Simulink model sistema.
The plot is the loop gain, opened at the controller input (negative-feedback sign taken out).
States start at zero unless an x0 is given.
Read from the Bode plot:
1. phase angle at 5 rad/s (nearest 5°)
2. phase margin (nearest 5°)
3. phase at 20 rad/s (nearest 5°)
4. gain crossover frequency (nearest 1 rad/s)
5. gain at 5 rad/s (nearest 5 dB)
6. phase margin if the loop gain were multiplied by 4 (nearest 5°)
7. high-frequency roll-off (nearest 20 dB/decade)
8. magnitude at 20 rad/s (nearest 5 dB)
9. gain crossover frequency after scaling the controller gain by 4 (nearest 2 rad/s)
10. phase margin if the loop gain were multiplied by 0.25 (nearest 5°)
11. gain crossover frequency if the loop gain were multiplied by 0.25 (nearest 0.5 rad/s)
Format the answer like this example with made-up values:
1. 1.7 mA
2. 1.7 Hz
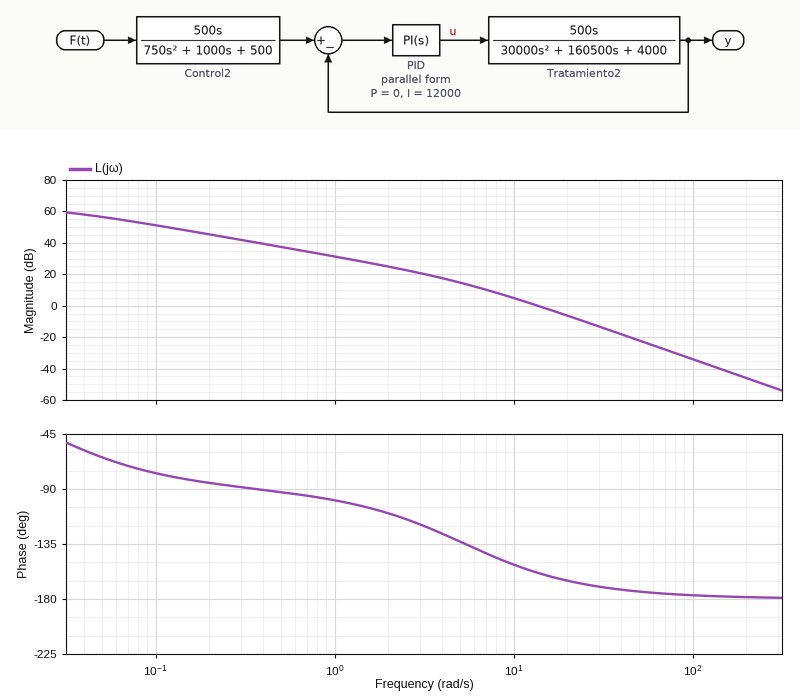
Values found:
1. -135°
2. 20°
3. -165°
4. 14 rad/s
5. 15 dB
6. 10°
7. -40 dB/decade
8. -5 dB
9. 28 rad/s
10. 40°
11. 6.0 rad/s
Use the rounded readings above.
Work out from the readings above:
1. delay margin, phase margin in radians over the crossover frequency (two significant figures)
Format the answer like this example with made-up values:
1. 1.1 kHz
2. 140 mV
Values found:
1. 0.025 s
